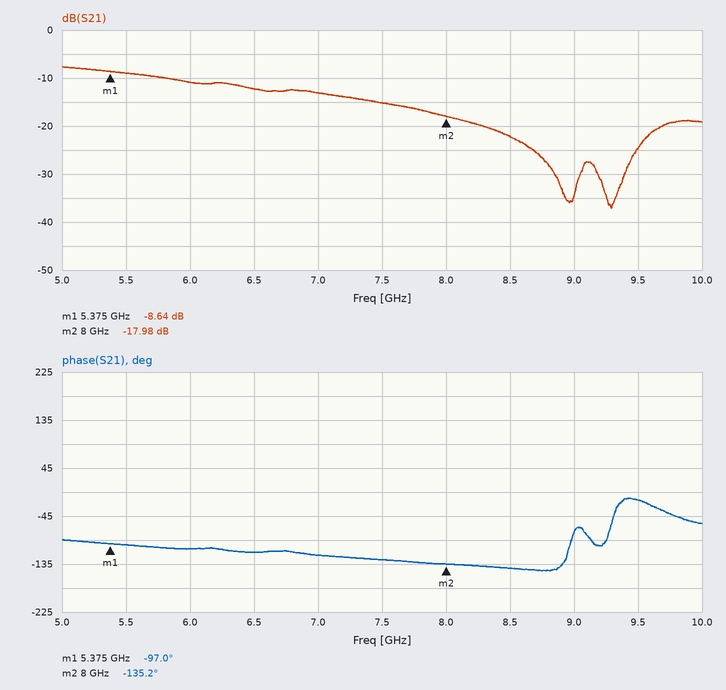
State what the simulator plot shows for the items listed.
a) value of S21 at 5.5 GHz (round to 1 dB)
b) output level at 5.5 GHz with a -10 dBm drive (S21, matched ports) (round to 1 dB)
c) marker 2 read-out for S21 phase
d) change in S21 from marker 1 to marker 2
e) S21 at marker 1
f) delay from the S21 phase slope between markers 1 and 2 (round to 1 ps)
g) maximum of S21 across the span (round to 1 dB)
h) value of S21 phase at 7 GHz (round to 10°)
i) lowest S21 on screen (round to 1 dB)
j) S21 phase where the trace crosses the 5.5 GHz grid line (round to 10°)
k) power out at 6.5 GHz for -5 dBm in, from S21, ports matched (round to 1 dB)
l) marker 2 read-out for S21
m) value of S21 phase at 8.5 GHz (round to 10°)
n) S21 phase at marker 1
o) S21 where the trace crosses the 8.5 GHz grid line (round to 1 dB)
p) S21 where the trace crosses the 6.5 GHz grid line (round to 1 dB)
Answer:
-9 dB
-19 dBm
-135.2°
-9.34 dB
-8.64 dB
40 ps
-8 dB
-120°
-37 dB
-100°
-17 dBm
-17.98 dB
-140°
-97.0°
-22 dB
-12 dB
